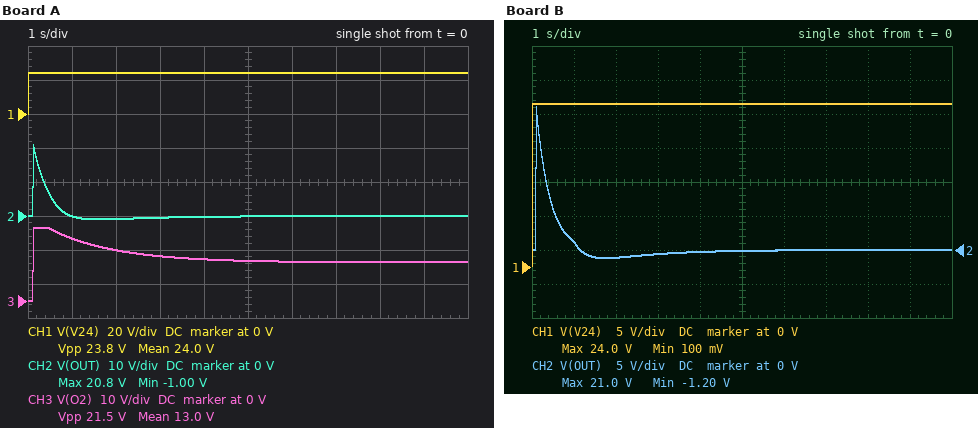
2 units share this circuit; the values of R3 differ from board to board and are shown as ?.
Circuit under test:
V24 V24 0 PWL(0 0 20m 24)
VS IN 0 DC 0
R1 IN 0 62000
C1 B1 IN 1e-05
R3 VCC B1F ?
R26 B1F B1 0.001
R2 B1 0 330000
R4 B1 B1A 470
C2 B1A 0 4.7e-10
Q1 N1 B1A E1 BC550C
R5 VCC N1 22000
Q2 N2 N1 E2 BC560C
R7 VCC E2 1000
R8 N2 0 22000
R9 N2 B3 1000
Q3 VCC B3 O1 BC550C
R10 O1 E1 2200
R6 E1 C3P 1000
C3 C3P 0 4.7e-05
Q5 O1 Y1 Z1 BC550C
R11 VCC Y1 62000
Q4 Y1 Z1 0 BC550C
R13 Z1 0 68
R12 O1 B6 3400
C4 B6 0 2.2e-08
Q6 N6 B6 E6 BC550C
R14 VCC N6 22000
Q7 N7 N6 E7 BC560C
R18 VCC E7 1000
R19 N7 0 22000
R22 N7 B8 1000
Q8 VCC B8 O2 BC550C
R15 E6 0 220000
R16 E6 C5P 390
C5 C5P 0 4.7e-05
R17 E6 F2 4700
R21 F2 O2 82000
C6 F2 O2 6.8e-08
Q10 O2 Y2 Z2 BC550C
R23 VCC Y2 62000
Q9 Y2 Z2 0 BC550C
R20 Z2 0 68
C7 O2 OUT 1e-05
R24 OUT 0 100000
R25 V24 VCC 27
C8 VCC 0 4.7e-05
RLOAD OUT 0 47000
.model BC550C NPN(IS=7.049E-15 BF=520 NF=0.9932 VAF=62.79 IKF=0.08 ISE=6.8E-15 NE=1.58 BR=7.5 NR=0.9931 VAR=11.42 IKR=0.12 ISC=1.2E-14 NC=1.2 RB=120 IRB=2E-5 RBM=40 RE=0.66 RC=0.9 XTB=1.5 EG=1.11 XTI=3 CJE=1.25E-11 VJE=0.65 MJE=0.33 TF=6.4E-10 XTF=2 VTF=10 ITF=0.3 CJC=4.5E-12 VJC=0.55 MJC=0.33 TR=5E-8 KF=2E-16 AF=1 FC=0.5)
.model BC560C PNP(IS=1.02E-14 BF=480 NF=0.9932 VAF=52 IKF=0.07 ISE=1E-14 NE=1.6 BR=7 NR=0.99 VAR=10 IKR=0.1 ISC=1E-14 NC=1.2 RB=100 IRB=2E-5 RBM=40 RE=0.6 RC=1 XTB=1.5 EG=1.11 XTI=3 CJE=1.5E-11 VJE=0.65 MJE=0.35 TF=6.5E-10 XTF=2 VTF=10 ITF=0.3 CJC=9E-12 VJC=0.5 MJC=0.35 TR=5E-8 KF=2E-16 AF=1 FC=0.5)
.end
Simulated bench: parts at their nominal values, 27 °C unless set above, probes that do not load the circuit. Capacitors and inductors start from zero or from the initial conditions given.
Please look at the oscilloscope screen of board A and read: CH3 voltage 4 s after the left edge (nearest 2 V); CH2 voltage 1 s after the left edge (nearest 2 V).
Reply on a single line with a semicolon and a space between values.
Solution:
12 V; 0 V
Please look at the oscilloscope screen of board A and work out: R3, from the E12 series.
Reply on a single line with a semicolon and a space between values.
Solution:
270 kΩ
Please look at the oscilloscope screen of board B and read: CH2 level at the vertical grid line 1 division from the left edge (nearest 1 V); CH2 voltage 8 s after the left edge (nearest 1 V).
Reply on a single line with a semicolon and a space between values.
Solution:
1 V; 0 V
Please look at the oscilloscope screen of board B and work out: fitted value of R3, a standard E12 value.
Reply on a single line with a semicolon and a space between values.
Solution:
220 kΩ
